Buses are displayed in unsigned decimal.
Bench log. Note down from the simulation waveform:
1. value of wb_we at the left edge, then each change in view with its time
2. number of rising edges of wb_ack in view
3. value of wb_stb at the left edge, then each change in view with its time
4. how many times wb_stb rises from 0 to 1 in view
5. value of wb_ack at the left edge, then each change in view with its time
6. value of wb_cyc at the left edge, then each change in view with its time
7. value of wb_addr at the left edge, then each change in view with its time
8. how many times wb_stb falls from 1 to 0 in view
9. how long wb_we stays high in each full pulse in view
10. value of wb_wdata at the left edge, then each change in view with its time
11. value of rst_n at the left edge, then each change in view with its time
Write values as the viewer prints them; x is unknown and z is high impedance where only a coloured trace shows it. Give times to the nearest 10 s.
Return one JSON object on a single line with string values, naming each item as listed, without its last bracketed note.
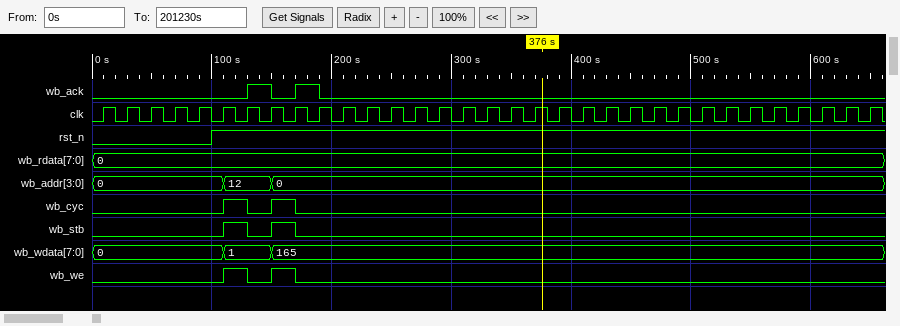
{"value of wb_we at the left edge, then each change in view with its time": "0, 1 at 110 s, 0 at 130 s, 1 at 150 s, 0 at 170 s", "number of rising edges of wb_ack in view": "2", "value of wb_stb at the left edge, then each change in view with its time": "0, 1 at 110 s, 0 at 130 s, 1 at 150 s, 0 at 170 s", "how many times wb_stb rises from 0 to 1 in view": "2", "value of wb_ack at the left edge, then each change in view with its time": "0, 1 at 130 s, 0 at 150 s, 1 at 170 s, 0 at 190 s", "value of wb_cyc at the left edge, then each change in view with its time": "0, 1 at 110 s, 0 at 130 s, 1 at 150 s, 0 at 170 s", "value of wb_addr at the left edge, then each change in view with its time": "0, 12 at 110 s, 0 at 150 s", "how many times wb_stb falls from 1 to 0 in view": "2", "how long wb_we stays high in each full pulse in view": "20 s, 20 s", "value of wb_wdata at the left edge, then each change in view with its time": "0, 1 at 110 s, 165 at 150 s", "value of rst_n at the left edge, then each change in view with its time": "0, 1 at 100 s"}
